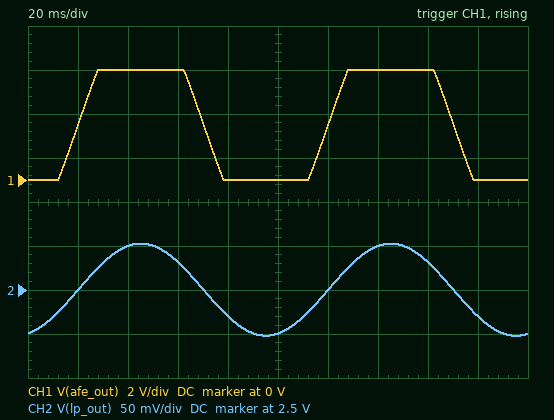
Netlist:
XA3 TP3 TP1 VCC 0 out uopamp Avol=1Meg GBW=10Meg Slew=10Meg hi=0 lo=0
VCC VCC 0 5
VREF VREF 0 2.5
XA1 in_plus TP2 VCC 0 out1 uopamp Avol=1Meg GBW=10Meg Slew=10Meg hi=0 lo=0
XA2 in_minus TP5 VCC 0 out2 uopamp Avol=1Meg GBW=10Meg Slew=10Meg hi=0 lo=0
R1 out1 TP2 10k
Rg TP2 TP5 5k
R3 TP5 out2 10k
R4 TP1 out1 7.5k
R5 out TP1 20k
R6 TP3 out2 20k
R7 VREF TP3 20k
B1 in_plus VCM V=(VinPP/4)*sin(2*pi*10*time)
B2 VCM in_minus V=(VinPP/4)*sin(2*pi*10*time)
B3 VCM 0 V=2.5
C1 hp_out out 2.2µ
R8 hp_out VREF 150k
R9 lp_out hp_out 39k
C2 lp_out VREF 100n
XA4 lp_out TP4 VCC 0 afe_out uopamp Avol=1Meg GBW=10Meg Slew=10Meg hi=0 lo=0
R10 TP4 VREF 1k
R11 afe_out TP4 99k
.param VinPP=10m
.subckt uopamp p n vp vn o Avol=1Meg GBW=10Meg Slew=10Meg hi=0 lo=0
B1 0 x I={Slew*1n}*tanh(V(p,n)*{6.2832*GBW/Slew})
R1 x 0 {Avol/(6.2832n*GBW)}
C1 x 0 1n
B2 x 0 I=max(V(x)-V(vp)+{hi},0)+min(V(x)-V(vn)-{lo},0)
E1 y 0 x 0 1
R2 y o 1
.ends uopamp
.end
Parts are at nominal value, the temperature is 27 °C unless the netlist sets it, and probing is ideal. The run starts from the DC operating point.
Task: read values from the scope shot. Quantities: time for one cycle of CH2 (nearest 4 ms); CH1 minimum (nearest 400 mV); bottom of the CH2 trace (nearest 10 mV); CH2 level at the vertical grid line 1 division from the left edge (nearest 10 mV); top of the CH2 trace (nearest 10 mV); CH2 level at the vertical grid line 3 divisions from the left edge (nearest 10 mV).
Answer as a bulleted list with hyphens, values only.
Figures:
- 100 ms
- 0 V
- 2.45 V
- 2.50 V
- 2.55 V
- 2.53 V
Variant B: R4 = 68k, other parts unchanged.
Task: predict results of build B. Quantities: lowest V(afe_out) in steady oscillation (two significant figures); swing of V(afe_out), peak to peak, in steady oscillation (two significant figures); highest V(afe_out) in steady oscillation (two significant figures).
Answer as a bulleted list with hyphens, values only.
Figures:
- 1.4 V
- 2.2 V
- 3.6 V
